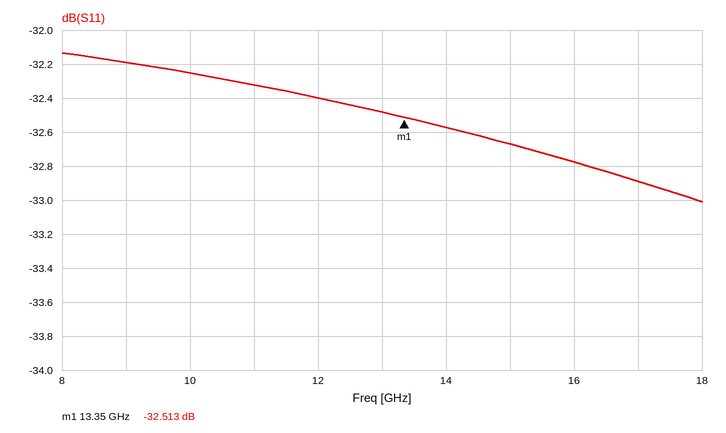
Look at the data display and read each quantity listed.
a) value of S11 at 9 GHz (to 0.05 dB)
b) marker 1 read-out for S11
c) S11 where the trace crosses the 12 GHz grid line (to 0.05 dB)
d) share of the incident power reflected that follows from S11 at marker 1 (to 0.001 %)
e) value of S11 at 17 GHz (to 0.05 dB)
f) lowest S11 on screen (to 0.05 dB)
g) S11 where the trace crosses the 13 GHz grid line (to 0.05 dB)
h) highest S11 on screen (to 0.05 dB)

-32.20 dB
-32.513 dB
-32.40 dB
0.056 %
-32.90 dB
-33.00 dB
-32.50 dB
-32.15 dB
